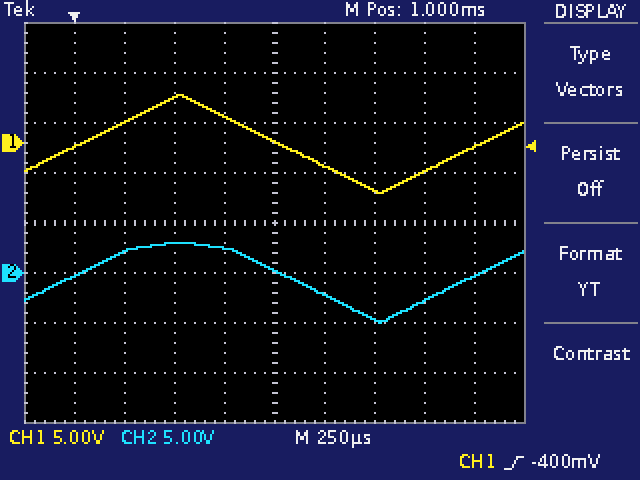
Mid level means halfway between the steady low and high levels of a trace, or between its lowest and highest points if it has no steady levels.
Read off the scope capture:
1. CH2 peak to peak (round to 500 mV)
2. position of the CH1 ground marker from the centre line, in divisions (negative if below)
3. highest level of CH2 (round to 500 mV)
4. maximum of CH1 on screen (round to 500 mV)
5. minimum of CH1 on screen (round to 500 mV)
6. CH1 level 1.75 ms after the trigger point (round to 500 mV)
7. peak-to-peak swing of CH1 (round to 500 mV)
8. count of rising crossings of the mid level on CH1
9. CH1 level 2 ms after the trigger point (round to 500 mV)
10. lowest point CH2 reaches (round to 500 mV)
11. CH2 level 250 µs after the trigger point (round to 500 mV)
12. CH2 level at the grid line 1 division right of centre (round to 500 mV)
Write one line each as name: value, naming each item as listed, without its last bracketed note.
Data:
CH2 peak to peak: 8.0 V
position of the CH1 ground marker from the centre line, in divisions: +1.6 div
highest level of CH2: 3.0 V
maximum of CH1 on screen: 5.0 V
minimum of CH1 on screen: -5.0 V
CH1 level 1.75 ms after the trigger point: -3.0 V
peak-to-peak swing of CH1: 10.0 V
count of rising crossings of the mid level on CH1: 2
CH1 level 2 ms after the trigger point: -500 mV
lowest point CH2 reaches: -5.0 V
CH2 level 250 µs after the trigger point: 2.0 V
CH2 level at the grid line 1 division right of centre: -2.0 V
